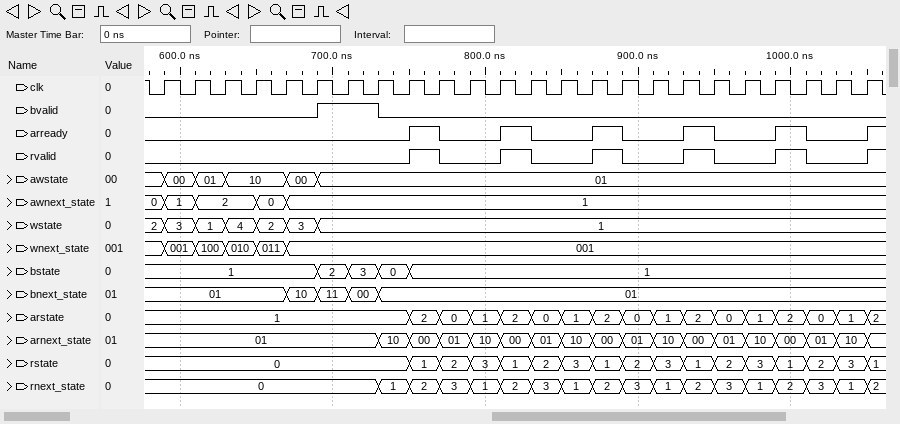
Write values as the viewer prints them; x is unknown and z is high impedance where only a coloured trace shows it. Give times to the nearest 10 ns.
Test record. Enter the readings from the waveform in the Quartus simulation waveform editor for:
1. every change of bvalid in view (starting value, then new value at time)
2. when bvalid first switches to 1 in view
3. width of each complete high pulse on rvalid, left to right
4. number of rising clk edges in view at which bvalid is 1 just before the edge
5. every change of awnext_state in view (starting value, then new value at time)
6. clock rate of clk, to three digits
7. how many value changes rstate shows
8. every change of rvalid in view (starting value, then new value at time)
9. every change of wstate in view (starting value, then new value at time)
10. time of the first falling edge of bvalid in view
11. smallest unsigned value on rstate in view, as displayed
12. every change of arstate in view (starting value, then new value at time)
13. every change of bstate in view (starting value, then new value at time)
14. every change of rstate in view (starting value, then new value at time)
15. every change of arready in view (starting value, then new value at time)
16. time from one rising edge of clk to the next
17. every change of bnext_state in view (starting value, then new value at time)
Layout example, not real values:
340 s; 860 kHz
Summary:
0, 1 at 690 ns, 0 at 730 ns; 690 ns; 20 ns, 20 ns, 20 ns, 20 ns, 20 ns; 2; 0, 1 at 590 ns, 2 at 610 ns, 0 at 650 ns, 1 at 670 ns; 50.0 MHz; 16; 0, 1 at 750 ns, 0 at 770 ns, 1 at 810 ns, 0 at 830 ns, 1 at 870 ns, 0 at 890 ns, 1 at 930 ns, 0 at 950 ns, 1 at 990 ns, 0 at 1010 ns, 1 at 1050 ns; 2, 3 at 590 ns, 1 at 610 ns, 4 at 630 ns, 2 at 650 ns, 3 at 670 ns, 1 at 690 ns; 730 ns; 0; 1, 2 at 750 ns, 0 at 770 ns, 1 at 790 ns, 2 at 810 ns, 0 at 830 ns, 1 at 850 ns, 2 at 870 ns, 0 at 890 ns, 1 at 910 ns, 2 at 930 ns, 0 at 950 ns, 1 at 970 ns, 2 at 990 ns, 0 at 1010 ns, 1 at 1030 ns, 2 at 1050 ns; 1, 2 at 690 ns, 3 at 710 ns, 0 at 730 ns, 1 at 750 ns; 0, 1 at 750 ns, 2 at 770 ns, 3 at 790 ns, 1 at 810 ns, 2 at 830 ns, 3 at 850 ns, 1 at 870 ns, 2 at 890 ns, 3 at 910 ns, 1 at 930 ns, 2 at 950 ns, 3 at 970 ns, 1 at 990 ns, 2 at 1010 ns, 3 at 1030 ns, 1 at 1050 ns; 0, 1 at 750 ns, 0 at 770 ns, 1 at 810 ns, 0 at 830 ns, 1 at 870 ns, 0 at 890 ns, 1 at 930 ns, 0 at 950 ns, 1 at 990 ns, 0 at 1010 ns, 1 at 1050 ns; 20 ns; 01, 10 at 670 ns, 11 at 690 ns, 00 at 710 ns, 01 at 730 ns
